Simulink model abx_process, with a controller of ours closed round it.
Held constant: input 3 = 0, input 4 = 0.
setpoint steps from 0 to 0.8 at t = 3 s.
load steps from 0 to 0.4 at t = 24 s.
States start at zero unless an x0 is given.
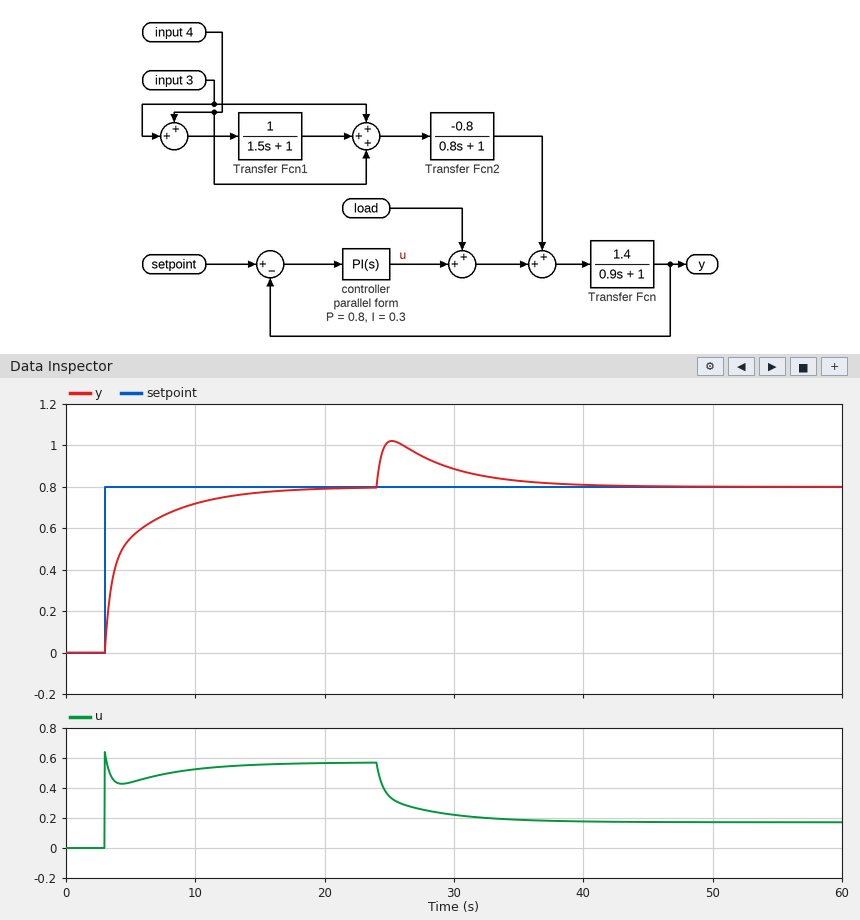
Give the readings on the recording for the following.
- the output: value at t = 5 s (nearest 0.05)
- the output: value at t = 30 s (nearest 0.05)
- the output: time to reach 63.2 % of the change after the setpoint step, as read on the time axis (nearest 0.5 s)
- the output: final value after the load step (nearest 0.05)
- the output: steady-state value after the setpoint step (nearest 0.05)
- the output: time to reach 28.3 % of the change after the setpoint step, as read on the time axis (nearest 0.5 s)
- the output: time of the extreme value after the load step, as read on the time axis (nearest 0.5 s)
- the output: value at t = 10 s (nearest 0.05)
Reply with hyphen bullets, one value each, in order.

- 0.55
- 0.90
- 4.5 s
- 0.80
- 0.80
- 3.5 s
- 25.0 s
- 0.70
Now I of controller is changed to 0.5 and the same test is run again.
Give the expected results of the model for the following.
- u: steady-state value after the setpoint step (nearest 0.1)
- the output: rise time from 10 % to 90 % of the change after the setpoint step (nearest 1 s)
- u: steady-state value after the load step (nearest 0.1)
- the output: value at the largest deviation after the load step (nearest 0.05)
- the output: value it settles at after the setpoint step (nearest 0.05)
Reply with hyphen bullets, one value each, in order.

- 0.6
- 4 s
- 0.2
- 1.00
- 0.80
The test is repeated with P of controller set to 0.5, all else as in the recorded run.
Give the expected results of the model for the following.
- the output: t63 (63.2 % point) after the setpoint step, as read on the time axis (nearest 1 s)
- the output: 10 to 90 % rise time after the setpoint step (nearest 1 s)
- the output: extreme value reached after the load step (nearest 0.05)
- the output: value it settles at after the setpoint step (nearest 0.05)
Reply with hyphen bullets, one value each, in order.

- 5 s
- 6 s
- 1.05
- 0.80
